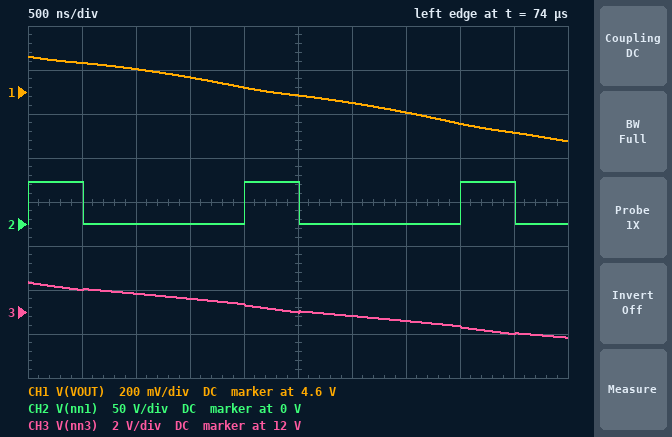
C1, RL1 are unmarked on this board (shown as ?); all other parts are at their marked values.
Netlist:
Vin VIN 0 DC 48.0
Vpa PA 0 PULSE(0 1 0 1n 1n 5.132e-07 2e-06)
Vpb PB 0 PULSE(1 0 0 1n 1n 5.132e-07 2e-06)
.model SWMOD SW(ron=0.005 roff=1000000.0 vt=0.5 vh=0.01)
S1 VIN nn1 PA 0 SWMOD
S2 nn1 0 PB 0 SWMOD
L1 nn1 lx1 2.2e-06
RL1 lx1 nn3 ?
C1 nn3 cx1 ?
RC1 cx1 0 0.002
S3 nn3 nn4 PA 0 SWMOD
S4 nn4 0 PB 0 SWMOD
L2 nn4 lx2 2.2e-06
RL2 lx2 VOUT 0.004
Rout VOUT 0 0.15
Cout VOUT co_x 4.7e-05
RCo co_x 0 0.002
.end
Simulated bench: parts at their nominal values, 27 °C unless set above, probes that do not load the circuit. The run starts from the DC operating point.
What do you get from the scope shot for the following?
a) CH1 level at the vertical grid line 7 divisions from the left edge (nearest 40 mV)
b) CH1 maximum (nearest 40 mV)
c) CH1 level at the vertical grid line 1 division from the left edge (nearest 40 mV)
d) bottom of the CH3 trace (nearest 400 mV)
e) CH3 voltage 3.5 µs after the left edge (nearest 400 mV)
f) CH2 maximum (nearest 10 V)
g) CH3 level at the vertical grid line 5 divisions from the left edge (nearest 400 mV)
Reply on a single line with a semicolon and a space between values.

4.52 V; 4.76 V; 4.72 V; 10.8 V; 11.6 V; 50 V; 12.0 V
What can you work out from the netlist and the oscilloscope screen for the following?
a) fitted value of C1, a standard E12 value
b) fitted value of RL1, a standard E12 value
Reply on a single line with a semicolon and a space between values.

120 µF; 0.01 Ω
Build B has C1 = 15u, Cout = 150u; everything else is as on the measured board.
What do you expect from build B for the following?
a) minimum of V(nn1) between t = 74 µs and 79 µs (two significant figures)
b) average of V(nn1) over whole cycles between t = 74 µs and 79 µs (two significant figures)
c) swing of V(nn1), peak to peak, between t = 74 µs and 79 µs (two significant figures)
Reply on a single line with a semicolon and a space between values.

-150 mV; 12 V; 48 V
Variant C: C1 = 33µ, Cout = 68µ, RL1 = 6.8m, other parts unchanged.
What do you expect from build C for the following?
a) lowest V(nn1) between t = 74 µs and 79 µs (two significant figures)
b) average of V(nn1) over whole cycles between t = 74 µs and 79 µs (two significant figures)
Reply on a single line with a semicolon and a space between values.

-90 mV; 12 V
